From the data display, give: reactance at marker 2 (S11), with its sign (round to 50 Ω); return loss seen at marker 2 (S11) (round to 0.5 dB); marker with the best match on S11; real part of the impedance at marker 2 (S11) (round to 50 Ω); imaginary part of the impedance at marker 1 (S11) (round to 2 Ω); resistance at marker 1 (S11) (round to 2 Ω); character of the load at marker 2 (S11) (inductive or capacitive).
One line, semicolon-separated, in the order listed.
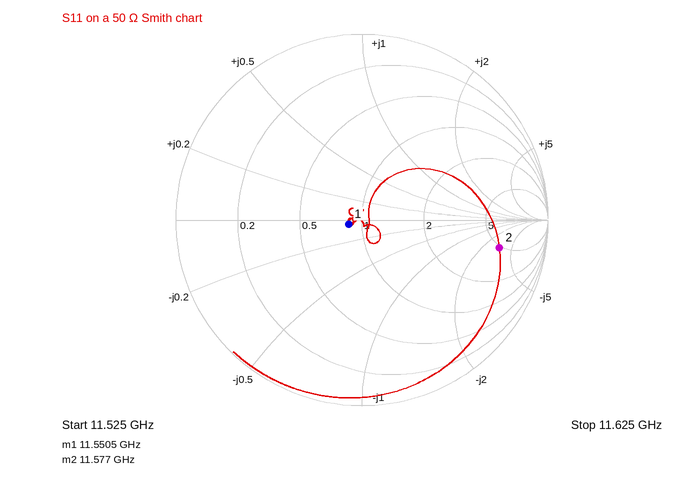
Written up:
-150 Ω; 2.5 dB; marker 1; 250 Ω; -2 Ω; 44 Ω; capacitive
